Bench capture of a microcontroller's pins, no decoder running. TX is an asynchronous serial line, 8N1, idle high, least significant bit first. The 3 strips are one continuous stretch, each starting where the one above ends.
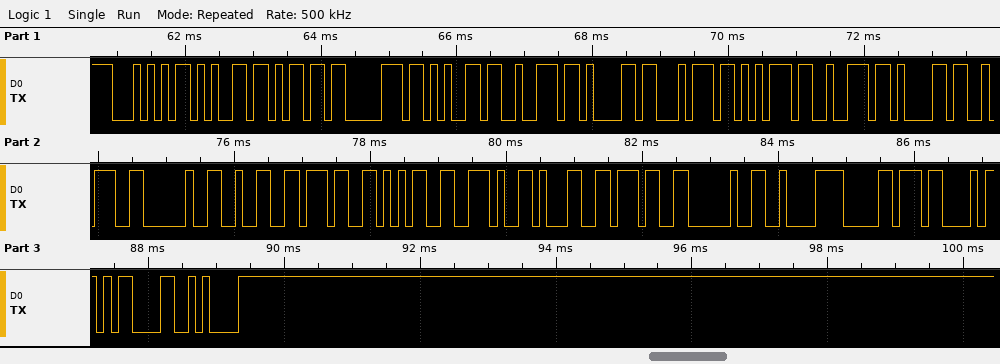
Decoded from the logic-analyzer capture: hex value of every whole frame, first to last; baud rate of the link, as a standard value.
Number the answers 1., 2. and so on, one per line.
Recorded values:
1. 54 65 6D 70 65 72 61 74 75 72 61 3A 20 32 37 35 2E 31 37 20 C2 B0 43 0D 0A
2. 9600 baud
